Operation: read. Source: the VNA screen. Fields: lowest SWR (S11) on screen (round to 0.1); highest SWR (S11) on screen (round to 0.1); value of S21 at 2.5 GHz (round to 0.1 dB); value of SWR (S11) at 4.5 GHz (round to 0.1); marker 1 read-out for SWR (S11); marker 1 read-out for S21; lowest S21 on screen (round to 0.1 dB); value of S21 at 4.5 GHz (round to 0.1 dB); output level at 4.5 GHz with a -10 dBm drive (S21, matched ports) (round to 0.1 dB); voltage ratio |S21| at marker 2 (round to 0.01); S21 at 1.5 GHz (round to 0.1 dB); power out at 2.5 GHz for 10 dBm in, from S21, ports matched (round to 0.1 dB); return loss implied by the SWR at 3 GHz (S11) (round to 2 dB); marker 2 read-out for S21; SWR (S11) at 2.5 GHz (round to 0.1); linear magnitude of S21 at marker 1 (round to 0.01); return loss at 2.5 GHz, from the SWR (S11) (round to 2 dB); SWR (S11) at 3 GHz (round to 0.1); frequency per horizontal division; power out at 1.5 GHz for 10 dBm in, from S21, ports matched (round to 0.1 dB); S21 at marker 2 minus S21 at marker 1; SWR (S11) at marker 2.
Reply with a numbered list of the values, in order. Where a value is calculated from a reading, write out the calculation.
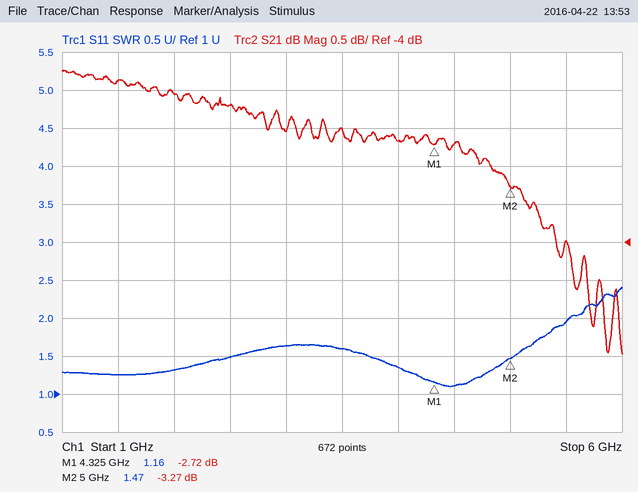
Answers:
1. 1.1
2. 2.4
3. -2.2 dB
4. 1.1
5. 1.16
6. -2.72 dB
7. -5.5 dB
8. -2.7 dB
9. -10 dBm + (-2.7 dB) = -12.7 dBm
10. 10^(-3.27/20) ≈ 0.69
11. -1.9 dB
12. 10 dBm + (-2.2 dB) = 7.8 dBm
13. −20 log10((1.6 − 1)/(1.6 + 1)) ≈ 12.7 dB, so 12 dB to the nearest 2 dB
14. -3.27 dB
15. 1.5
16. 10^(-2.72/20) ≈ 0.73
17. −20 log10((1.5 − 1)/(1.5 + 1)) ≈ 14 dB
18. 1.6
19. 500 MHz
20. 10 dBm + (-1.9 dB) = 8.1 dBm
21. -3.27 − (-2.72) = -0.55 dB
22. 1.47
